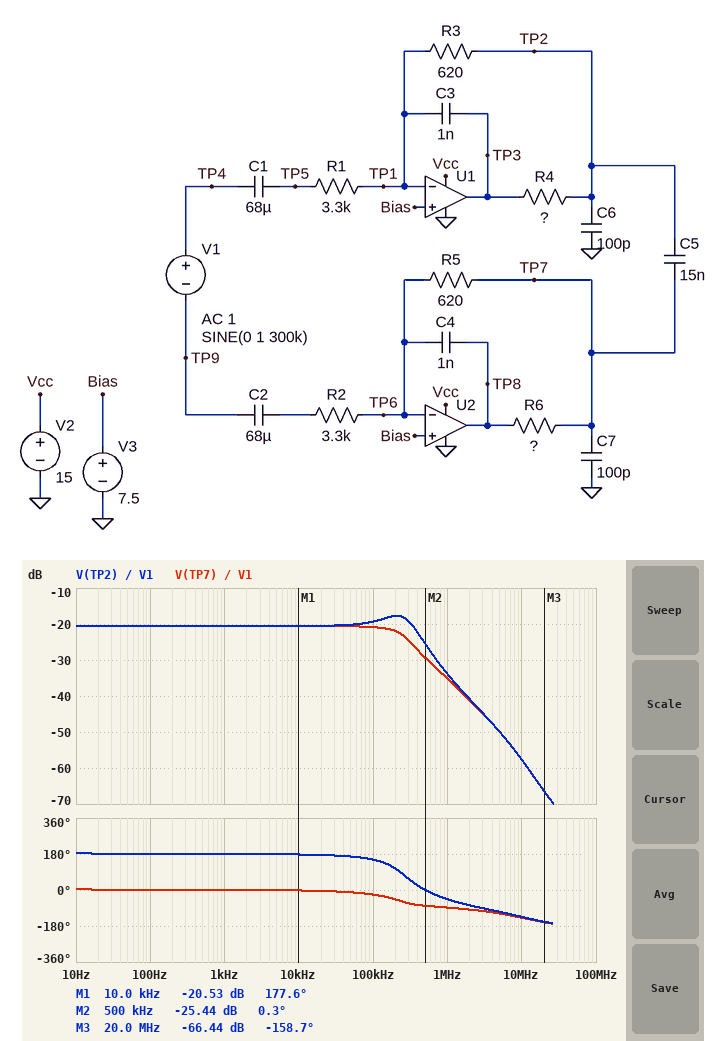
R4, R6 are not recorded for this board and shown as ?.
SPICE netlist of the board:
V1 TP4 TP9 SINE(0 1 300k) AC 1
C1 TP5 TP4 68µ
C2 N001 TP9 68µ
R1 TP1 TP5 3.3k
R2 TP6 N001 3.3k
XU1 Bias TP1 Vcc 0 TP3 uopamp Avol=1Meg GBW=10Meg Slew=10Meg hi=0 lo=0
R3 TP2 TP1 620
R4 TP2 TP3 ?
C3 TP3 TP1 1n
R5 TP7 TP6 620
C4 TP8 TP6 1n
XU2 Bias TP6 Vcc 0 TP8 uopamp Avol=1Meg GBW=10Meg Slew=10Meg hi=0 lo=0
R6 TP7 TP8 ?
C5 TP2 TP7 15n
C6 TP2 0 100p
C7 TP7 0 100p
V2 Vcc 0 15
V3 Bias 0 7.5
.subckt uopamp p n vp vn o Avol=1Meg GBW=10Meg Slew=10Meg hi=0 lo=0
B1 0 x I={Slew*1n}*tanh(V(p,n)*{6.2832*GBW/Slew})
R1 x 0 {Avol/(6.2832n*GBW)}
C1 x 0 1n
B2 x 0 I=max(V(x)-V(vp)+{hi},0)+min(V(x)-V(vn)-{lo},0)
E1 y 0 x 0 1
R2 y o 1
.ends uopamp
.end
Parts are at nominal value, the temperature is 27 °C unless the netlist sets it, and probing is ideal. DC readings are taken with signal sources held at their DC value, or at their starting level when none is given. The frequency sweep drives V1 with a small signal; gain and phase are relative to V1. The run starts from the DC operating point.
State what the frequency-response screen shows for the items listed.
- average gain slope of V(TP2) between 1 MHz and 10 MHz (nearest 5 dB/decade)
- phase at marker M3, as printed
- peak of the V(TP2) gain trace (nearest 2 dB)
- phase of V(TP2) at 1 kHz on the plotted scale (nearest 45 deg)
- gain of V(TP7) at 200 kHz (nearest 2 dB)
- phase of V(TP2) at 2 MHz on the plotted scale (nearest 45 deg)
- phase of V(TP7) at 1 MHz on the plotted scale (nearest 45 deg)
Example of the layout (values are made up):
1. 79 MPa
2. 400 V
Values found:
1. -25 dB/decade
2. -158.7 deg
3. -18 dB
4. 180 deg
5. -22 dB
6. -90 deg
7. -90 deg
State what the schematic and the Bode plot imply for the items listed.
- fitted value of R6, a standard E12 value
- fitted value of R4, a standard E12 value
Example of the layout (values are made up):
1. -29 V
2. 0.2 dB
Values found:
1. 4.7 Ω
2. 33 Ω
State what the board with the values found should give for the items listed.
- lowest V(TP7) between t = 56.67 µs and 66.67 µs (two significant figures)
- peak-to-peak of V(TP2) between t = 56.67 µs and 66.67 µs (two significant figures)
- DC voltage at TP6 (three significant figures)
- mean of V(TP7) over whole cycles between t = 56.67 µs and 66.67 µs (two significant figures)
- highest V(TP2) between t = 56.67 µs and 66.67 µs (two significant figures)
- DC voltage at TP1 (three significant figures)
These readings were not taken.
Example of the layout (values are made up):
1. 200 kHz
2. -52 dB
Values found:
1. 7.4 V
2. 220 mV
3. 7.50 V
4. 7.5 V
5. 7.6 V
6. 7.50 V
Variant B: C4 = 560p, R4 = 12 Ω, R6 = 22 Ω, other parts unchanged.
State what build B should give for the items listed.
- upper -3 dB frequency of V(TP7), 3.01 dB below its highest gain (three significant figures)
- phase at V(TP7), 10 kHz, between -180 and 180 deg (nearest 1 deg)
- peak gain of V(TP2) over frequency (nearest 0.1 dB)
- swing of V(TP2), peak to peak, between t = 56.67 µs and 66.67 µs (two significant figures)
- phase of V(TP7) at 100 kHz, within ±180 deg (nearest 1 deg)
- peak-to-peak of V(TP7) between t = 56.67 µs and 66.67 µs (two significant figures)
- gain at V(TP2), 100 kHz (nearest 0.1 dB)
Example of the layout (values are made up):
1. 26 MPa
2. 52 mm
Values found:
1. 408 kHz
2. -1 deg
3. -20.2 dB
4. 180 mV
5. -15 deg
6. 230 mV
7. -20.4 dB
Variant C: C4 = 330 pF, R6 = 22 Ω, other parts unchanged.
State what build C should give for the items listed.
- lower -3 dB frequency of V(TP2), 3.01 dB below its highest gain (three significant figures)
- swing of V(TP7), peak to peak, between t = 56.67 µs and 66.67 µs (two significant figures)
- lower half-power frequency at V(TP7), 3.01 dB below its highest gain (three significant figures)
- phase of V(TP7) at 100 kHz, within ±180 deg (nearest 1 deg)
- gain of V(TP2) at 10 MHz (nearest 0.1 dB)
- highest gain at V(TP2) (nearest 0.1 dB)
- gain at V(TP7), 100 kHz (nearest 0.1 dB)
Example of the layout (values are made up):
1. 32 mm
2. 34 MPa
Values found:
1. 108 kHz
2. 190 mV
3. 1.06 Hz
4. -9 deg
5. -53.0 dB
6. -16.0 dB
7. -20.1 dB
